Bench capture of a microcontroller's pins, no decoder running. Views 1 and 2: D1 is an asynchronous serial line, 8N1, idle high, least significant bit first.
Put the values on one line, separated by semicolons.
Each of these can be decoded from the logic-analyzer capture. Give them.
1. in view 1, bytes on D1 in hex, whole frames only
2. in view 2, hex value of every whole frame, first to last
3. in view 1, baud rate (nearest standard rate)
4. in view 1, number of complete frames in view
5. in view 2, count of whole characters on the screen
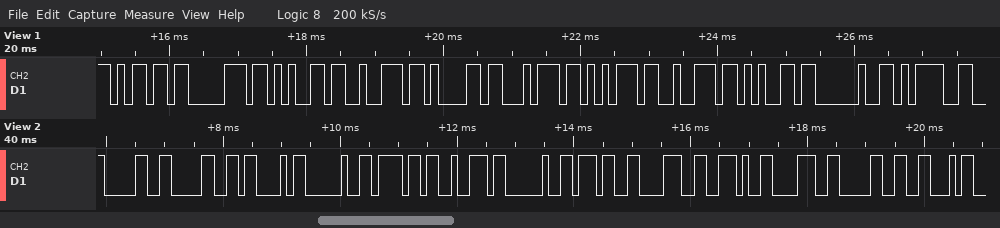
6D 70 65 72 61 74 75 72 65 20 3D; 30 30 43 20 6F 72 20 37 38 2E 38 30 46; 9600 baud; 11; 13
